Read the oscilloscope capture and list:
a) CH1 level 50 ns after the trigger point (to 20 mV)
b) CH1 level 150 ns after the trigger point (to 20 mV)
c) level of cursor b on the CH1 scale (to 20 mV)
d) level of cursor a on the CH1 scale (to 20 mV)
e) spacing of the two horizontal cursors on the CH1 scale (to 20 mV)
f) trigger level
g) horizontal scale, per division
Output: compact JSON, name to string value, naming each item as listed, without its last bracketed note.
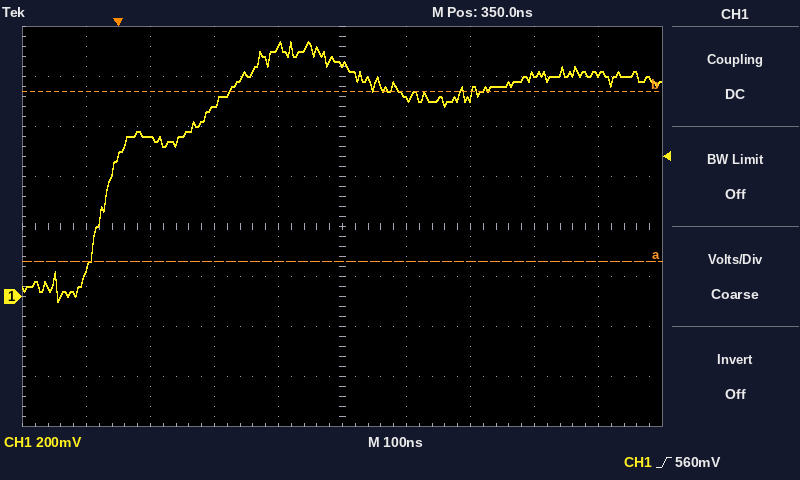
{"CH1 level 50 ns after the trigger point": "640 mV", "CH1 level 150 ns after the trigger point": "760 mV", "level of cursor b on the CH1 scale": "820 mV", "level of cursor a on the CH1 scale": "140 mV", "spacing of the two horizontal cursors on the CH1 scale": "680 mV", "trigger level": "560 mV", "horizontal scale, per division": "100 ns"}
